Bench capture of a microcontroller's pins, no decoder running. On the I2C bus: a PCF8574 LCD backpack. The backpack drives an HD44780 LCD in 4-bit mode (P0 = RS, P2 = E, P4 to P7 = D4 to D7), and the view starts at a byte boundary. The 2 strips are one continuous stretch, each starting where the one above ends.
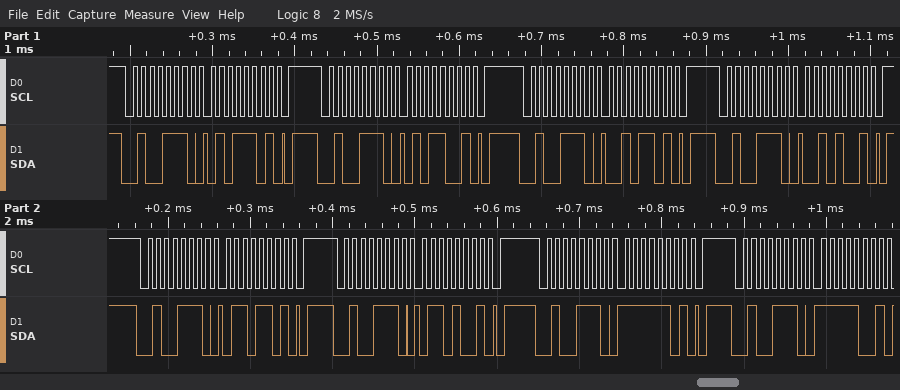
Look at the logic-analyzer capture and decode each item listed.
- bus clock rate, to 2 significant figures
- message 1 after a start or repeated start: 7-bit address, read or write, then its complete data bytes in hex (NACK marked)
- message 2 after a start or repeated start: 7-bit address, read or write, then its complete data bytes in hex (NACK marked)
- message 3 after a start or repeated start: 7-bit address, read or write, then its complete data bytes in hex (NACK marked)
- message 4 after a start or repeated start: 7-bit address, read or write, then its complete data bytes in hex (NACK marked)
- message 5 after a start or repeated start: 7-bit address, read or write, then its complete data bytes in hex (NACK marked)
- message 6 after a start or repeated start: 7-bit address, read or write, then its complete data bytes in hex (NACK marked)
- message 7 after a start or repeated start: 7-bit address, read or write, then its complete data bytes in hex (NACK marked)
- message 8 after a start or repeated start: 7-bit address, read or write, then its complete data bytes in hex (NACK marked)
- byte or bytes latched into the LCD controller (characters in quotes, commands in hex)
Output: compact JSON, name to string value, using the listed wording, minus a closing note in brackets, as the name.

{"bus clock rate, to 2 significant figures": "100 kHz", "message 1 after a start or repeated start: 7-bit address, read or write, then its complete data bytes in hex": "0x27 write: 5D", "message 2 after a start or repeated start: 7-bit address, read or write, then its complete data bytes in hex": "0x27 write: 59", "message 3 after a start or repeated start: 7-bit address, read or write, then its complete data bytes in hex": "0x27 write: 2D", "message 4 after a start or repeated start: 7-bit address, read or write, then its complete data bytes in hex": "0x27 write: 29", "message 5 after a start or repeated start: 7-bit address, read or write, then its complete data bytes in hex": "0x27 write: 6D", "message 6 after a start or repeated start: 7-bit address, read or write, then its complete data bytes in hex": "0x27 write: 69", "message 7 after a start or repeated start: 7-bit address, read or write, then its complete data bytes in hex": "0x27 write: FD", "message 8 after a start or repeated start: 7-bit address, read or write, then its complete data bytes in hex": "0x27 write: F9", "byte or bytes latched into the LCD controller": "'R' 'o'"}
